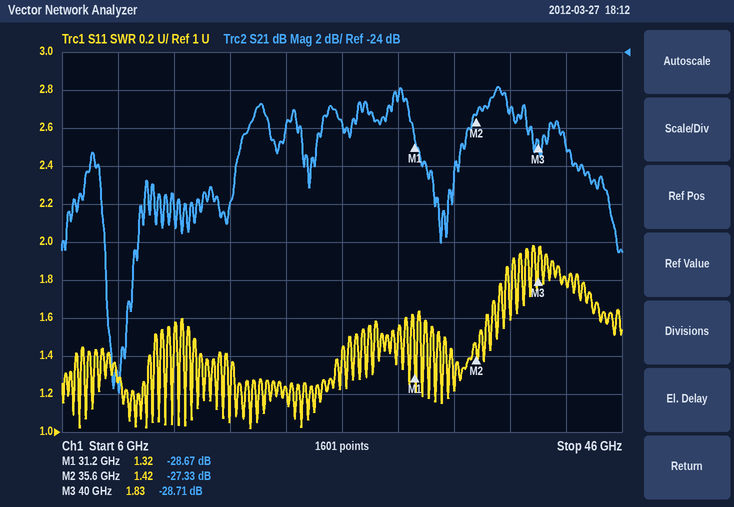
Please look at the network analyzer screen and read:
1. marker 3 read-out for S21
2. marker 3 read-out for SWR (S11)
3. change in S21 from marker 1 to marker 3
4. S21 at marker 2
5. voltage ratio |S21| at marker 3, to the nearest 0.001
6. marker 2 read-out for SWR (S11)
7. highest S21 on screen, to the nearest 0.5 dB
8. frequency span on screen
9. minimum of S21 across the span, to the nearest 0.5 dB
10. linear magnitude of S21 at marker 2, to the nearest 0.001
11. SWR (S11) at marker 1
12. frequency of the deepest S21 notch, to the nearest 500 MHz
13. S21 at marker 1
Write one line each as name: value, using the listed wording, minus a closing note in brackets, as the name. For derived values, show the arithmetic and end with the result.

marker 3 read-out for S21: -28.71 dB
marker 3 read-out for SWR: 1.83
change in S21 from marker 1 to marker 3: -28.71 − (-28.67) = -0.04 dB
S21 at marker 2: -27.33 dB
voltage ratio |S21| at marker 3, to the nearest 0.001: 10^(-28.71/20) ≈ 0.037
marker 2 read-out for SWR: 1.42
highest S21 on screen, to the nearest 0.5 dB: -26.0 dB
frequency span on screen: 40 GHz
minimum of S21 across the span, to the nearest 0.5 dB: -42.0 dB
linear magnitude of S21 at marker 2, to the nearest 0.001: 10^(-27.33/20) ≈ 0.043
SWR (S11) at marker 1: 1.32
frequency of the deepest S21 notch, to the nearest 500 MHz: 10.0 GHz
S21 at marker 1: -28.67 dB
